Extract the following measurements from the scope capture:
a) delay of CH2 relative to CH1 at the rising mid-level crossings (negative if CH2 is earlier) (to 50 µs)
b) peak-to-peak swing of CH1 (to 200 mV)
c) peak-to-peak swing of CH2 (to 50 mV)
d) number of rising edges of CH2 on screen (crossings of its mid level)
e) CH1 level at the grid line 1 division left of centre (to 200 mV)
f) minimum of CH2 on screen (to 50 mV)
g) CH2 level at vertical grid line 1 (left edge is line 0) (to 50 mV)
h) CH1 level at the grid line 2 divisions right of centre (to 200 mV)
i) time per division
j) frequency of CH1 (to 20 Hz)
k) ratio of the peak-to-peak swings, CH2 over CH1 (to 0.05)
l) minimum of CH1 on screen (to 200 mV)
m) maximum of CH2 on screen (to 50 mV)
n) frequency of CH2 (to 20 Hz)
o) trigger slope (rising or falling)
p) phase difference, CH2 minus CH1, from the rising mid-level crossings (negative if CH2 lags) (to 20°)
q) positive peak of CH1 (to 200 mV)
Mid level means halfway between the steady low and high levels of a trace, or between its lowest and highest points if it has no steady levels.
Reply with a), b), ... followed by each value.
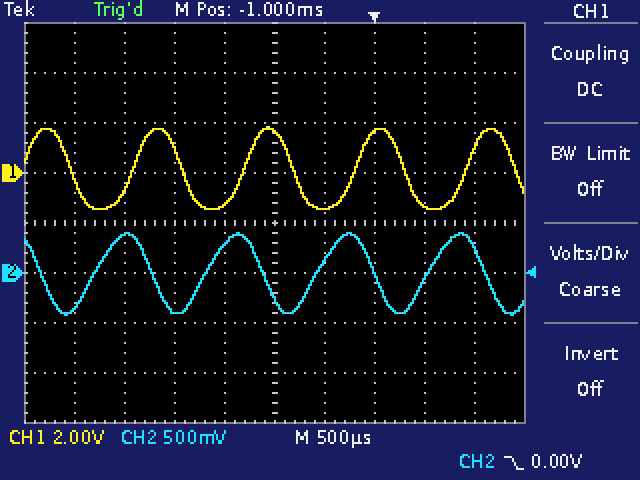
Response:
a) -400 µs
b) 3.2 V
c) 800 mV
d) 4
e) -1.2 V
f) -400 mV
g) -350 mV
h) 1.6 V
i) 500 µs
j) 900 Hz
k) 0.25
l) -1.4 V
m) 400 mV
n) 900 Hz
o) falling
p) +120°
q) 1.8 V
